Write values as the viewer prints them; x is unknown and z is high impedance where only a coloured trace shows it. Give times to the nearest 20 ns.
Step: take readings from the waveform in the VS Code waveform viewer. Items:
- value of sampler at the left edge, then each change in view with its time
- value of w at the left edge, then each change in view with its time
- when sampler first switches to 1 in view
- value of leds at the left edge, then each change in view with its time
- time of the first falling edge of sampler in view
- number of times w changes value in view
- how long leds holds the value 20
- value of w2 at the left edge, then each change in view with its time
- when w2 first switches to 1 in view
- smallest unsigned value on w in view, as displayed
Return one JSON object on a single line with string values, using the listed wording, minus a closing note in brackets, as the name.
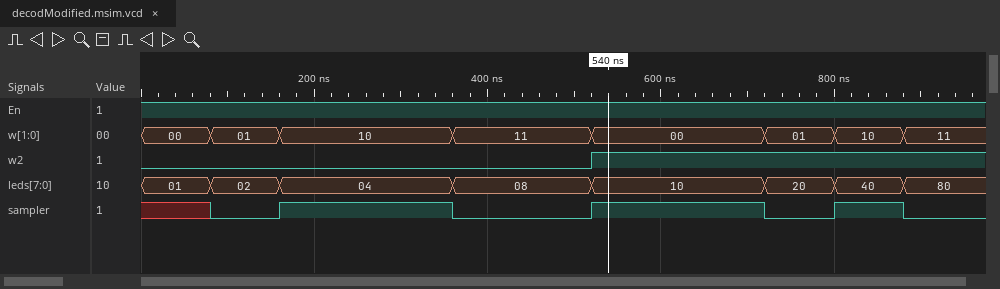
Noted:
{"value of sampler at the left edge, then each change in view with its time": "x, 0 at 80 ns, 1 at 160 ns, 0 at 360 ns, 1 at 520 ns, 0 at 720 ns, 1 at 800 ns, 0 at 880 ns", "value of w at the left edge, then each change in view with its time": "00, 01 at 80 ns, 10 at 160 ns, 11 at 360 ns, 00 at 520 ns, 01 at 720 ns, 10 at 800 ns, 11 at 880 ns", "when sampler first switches to 1 in view": "160 ns", "value of leds at the left edge, then each change in view with its time": "01, 02 at 80 ns, 04 at 160 ns, 08 at 360 ns, 10 at 520 ns, 20 at 720 ns, 40 at 800 ns, 80 at 880 ns", "time of the first falling edge of sampler in view": "360 ns", "number of times w changes value in view": "7", "how long leds holds the value 20": "80 ns", "value of w2 at the left edge, then each change in view with its time": "0, 1 at 520 ns", "when w2 first switches to 1 in view": "520 ns", "smallest unsigned value on w in view, as displayed": "00"}
